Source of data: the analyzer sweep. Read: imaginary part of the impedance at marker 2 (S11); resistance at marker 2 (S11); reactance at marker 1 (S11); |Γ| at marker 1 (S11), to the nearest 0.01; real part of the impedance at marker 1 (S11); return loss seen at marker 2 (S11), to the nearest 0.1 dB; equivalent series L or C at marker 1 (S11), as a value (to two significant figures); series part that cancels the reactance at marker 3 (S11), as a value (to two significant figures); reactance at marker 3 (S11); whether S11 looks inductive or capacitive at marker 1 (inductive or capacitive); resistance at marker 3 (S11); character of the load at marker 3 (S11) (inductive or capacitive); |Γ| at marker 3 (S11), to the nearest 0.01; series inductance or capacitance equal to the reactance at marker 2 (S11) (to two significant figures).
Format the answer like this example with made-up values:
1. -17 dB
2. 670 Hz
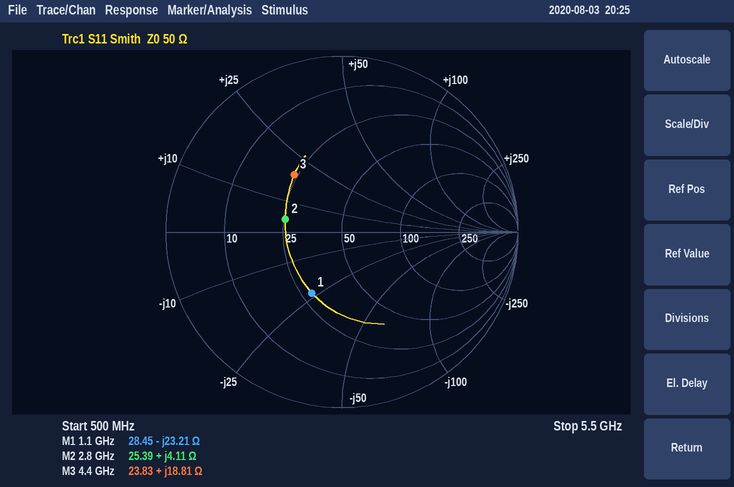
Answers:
1. +4.11 Ω
2. 25.39 Ω
3. -23.21 Ω
4. 0.39
5. 28.45 Ω
6. 9.6 dB
7. 6.2 pF
8. 1.9 pF
9. +18.81 Ω
10. capacitive
11. 23.83 Ω
12. inductive
13. 0.42
14. 230 pH
